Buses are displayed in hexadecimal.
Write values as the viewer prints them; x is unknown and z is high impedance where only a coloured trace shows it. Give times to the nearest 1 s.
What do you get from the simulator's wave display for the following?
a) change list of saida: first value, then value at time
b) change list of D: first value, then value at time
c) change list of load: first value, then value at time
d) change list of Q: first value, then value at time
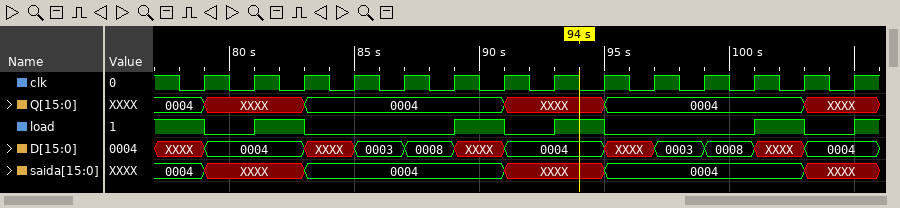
0004, XXXX at 79 s, 0004 at 83 s, XXXX at 91 s, 0004 at 95 s, XXXX at 103 s
XXXX, 0004 at 79 s, XXXX at 83 s, 0003 at 85 s, 0008 at 87 s, XXXX at 89 s, 0004 at 91 s, XXXX at 95 s, 0003 at 97 s, 0008 at 99 s, XXXX at 101 s, 0004 at 103 s
1, 0 at 79 s, 1 at 81 s, 0 at 83 s, 1 at 89 s, 0 at 91 s, 1 at 93 s, 0 at 95 s, 1 at 101 s, 0 at 103 s, 1 at 105 s
0004, XXXX at 79 s, 0004 at 83 s, XXXX at 91 s, 0004 at 95 s, XXXX at 103 s
